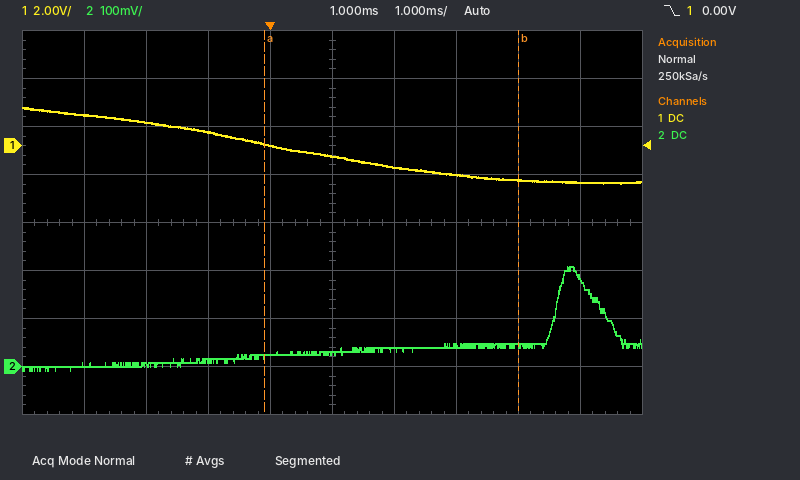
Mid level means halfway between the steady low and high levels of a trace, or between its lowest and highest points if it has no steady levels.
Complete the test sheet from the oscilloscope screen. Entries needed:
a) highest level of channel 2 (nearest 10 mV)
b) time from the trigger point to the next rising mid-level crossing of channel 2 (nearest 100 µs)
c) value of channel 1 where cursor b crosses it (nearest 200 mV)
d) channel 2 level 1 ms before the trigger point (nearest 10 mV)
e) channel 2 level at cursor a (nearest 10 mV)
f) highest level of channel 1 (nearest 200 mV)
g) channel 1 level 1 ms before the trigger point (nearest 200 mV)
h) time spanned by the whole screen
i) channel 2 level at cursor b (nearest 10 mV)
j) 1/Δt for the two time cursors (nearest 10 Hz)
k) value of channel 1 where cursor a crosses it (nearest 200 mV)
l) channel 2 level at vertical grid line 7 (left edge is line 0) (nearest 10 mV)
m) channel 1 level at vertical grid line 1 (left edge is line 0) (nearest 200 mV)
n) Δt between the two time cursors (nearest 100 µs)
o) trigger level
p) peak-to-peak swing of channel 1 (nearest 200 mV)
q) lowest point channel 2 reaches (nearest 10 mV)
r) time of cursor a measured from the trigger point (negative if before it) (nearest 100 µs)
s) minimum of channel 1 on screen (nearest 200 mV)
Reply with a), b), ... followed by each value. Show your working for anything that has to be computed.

a) 210 mV
b) 4.6 ms
c) -1.4 V
d) 10 mV
e) 20 mV
f) 1.6 V
g) 600 mV
h) 10 ms
i) 40 mV
j) 1 / 4.1 ms ≈ 240 Hz
k) 0.0 V
l) 40 mV
m) 1.2 V
n) 4.1 ms
o) 0.00 V
p) 1.6 V − (-1.6 V) = 3.2 V
q) -10 mV
r) -100 µs
s) -1.6 V
